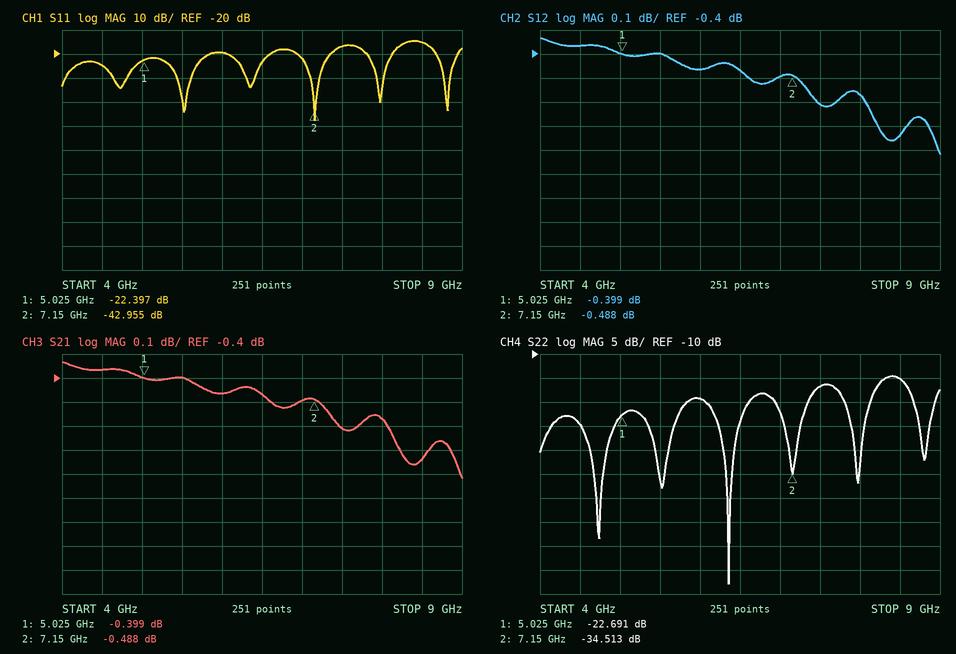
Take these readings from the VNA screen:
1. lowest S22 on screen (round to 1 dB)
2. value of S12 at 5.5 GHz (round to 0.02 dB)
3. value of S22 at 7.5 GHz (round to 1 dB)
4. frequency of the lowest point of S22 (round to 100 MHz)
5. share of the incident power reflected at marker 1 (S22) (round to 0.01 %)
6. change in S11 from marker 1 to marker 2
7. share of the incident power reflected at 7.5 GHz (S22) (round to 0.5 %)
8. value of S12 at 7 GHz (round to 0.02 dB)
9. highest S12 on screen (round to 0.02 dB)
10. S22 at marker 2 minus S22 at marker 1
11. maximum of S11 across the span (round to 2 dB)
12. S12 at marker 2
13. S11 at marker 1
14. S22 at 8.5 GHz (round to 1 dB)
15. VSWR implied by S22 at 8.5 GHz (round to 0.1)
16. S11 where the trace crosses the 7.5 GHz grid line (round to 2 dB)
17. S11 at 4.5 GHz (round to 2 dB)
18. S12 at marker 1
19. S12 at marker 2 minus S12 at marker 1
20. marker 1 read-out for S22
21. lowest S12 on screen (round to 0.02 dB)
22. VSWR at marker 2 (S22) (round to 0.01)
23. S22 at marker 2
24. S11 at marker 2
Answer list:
-58 dB
-0.40 dB
-17 dB
6.4 GHz
0.54 %
-20.558 dB
2.0 %
-0.50 dB
-0.34 dB
-11.822 dB
-14 dB
-0.488 dB
-22.397 dB
-15 dB
1.4
-16 dB
-24 dB
-0.399 dB
-0.089 dB
-22.691 dB
-0.82 dB
1.04
-34.513 dB
-42.955 dB
